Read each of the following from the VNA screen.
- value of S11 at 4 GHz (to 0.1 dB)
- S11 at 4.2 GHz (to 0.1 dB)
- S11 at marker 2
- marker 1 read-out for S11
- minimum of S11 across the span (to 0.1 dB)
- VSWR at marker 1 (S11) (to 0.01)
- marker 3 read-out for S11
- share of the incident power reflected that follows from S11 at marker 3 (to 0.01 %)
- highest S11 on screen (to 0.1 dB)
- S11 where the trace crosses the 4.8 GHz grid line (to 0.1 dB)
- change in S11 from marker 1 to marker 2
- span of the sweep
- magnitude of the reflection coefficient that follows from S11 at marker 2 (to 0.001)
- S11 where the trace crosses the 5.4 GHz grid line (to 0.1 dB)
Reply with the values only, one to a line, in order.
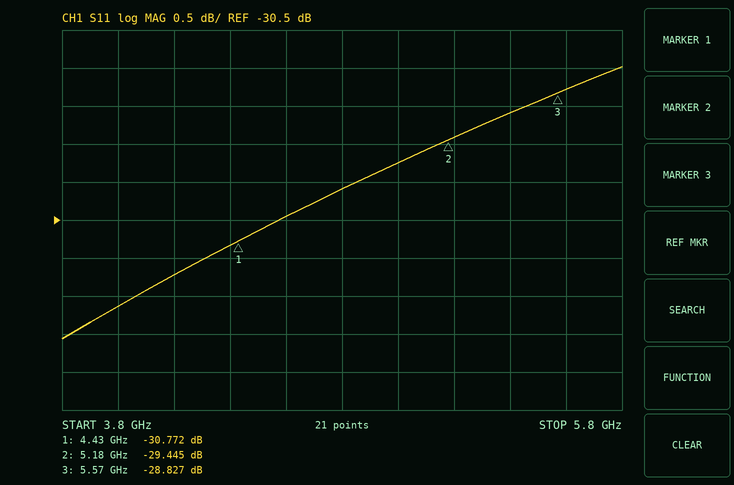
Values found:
-31.6 dB
-31.2 dB
-29.445 dB
-30.772 dB
-32.1 dB
1.06
-28.827 dB
0.13 %
-28.5 dB
-30.1 dB
1.327 dB
2 GHz
0.034
-29.1 dB
